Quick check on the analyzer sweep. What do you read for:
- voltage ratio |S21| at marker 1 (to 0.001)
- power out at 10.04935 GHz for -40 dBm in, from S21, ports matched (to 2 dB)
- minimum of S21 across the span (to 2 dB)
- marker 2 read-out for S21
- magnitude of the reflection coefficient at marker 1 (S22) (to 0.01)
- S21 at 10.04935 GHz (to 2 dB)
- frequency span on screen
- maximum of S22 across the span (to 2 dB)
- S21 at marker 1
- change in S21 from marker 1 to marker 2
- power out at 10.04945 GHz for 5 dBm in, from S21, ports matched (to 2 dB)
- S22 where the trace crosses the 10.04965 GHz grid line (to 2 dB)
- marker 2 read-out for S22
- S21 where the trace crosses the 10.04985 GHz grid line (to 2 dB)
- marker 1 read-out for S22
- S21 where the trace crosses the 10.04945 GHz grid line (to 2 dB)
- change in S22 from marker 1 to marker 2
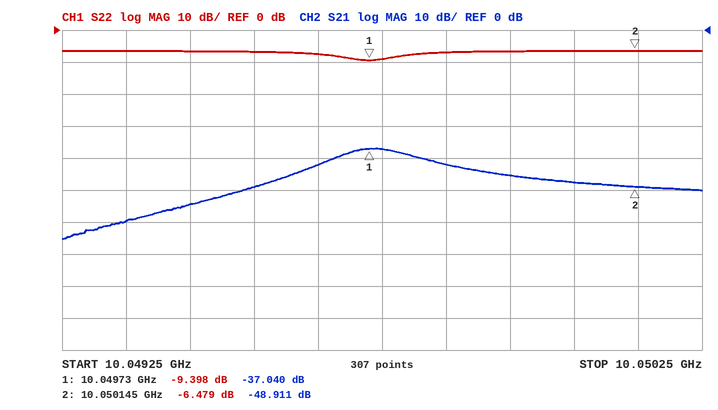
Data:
0.014
-100 dBm
-66 dB
-48.911 dB
0.34
-60 dB
1 MHz
-6 dB
-37.040 dB
-11.871 dB
-50 dBm
-8 dB
-6.479 dB
-42 dB
-9.398 dB
-54 dB
2.919 dB
